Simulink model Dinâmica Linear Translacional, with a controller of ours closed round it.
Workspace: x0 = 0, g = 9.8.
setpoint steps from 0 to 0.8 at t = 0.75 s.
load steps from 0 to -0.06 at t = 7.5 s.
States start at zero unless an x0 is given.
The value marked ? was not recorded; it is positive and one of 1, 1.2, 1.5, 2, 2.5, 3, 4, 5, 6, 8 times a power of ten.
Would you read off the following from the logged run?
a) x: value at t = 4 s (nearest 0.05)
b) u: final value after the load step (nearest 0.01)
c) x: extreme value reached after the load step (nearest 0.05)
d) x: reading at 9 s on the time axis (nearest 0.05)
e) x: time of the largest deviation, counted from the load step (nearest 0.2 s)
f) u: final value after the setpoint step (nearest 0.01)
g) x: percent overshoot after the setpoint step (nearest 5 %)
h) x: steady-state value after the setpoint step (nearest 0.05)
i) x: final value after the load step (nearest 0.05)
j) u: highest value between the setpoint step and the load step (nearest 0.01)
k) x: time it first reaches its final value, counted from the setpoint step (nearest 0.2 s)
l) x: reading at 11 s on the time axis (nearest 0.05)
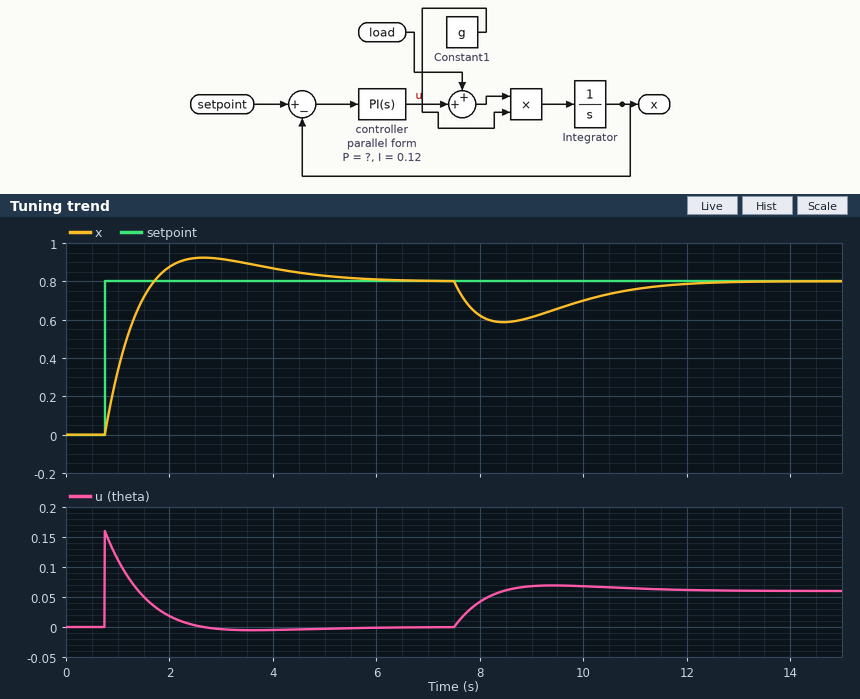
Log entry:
0.85
0.06
0.60
0.60
1.0 s
0.00
15 %
0.80
0.80
0.16
1.0 s
0.75
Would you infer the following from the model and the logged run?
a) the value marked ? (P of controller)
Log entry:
0.2
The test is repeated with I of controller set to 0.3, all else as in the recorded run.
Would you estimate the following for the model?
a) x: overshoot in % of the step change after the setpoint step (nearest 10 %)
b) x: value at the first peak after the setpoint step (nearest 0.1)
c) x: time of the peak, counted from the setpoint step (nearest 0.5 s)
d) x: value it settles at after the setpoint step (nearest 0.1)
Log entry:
30 %
1.0
1.5 s
0.8
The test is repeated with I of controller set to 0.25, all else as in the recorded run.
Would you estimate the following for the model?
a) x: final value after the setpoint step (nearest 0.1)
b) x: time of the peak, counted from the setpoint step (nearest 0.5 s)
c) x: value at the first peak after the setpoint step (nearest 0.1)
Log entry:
0.8
1.5 s
1.0
